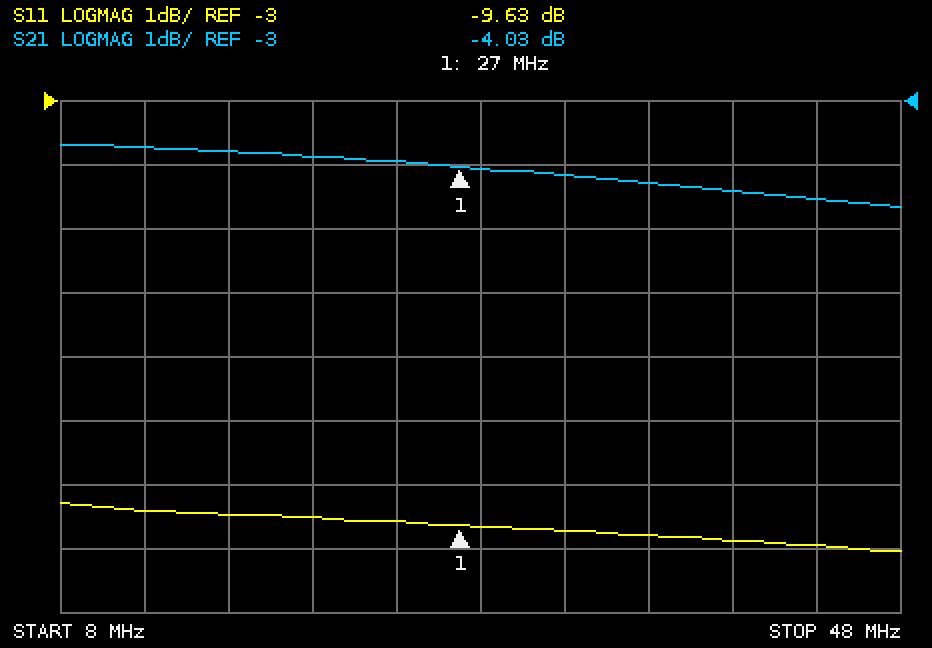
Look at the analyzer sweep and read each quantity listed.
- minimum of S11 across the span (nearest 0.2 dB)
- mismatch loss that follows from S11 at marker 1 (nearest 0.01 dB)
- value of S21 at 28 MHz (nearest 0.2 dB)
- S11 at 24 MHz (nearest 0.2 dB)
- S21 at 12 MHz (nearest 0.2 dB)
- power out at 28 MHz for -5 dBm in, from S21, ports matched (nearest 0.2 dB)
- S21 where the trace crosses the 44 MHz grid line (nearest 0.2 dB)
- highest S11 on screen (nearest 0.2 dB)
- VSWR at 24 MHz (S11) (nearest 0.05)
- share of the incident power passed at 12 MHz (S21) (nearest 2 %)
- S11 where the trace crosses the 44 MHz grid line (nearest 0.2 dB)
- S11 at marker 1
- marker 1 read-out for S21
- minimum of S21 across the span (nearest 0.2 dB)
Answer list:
-10.0 dB
0.50 dB
-4.0 dB
-9.6 dB
-3.8 dB
-9.0 dBm
-4.6 dB
-9.2 dB
2.00
42 %
-10.0 dB
-9.63 dB
-4.03 dB
-4.6 dB
